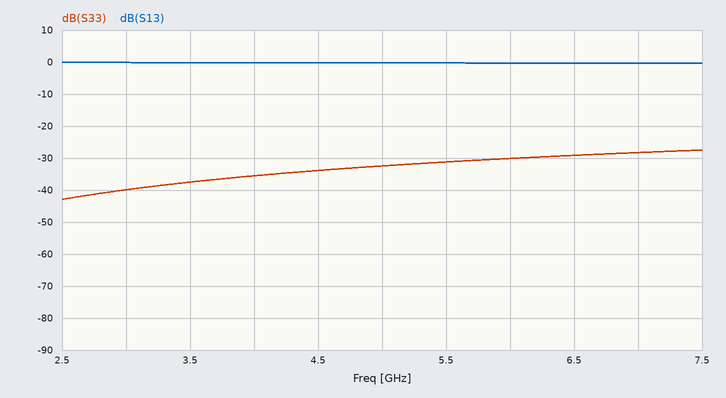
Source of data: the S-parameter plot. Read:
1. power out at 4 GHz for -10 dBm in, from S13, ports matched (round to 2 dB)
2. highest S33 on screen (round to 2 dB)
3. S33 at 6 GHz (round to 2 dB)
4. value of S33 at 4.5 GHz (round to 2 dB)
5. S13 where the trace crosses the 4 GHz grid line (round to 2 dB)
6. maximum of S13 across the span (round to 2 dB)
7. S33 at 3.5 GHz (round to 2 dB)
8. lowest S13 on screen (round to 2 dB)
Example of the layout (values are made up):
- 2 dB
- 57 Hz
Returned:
- -10 dBm
- -28 dB
- -30 dB
- -34 dB
- 0 dB
- 0 dB
- -38 dB
- 0 dB
